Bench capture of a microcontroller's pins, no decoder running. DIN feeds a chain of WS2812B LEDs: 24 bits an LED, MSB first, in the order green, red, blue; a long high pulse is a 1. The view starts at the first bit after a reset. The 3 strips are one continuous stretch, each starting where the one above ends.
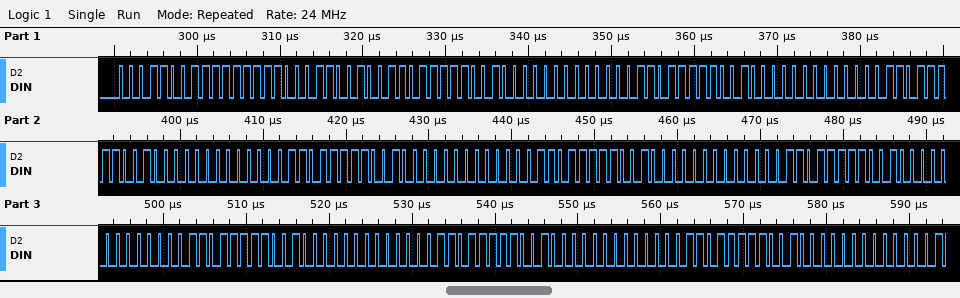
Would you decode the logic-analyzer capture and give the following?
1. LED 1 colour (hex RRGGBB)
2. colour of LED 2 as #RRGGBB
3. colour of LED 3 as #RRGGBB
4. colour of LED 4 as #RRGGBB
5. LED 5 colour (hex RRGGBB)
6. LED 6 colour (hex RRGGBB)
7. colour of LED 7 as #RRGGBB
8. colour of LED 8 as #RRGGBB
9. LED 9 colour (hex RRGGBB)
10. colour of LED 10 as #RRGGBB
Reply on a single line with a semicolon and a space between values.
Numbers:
#FF1919; #C83700; #C83700; #C83700; #C83700; #C83700; #C83700; #C83700; #C83700; #C83700
